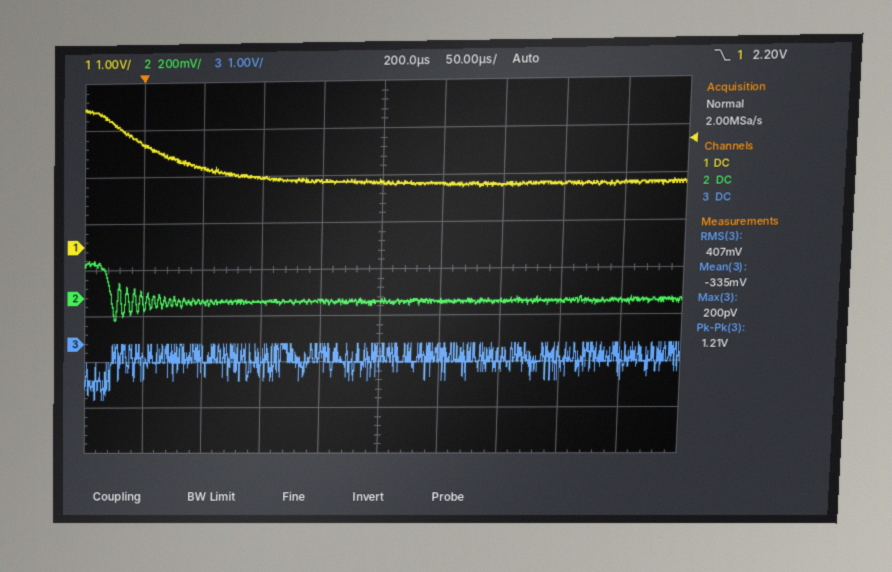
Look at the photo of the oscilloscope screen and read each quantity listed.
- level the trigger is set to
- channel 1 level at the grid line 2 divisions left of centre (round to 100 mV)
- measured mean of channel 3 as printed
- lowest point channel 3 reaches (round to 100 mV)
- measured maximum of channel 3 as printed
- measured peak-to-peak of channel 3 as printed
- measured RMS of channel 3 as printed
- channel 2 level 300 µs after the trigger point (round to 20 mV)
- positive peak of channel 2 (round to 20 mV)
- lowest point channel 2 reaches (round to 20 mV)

2.20 V
1.5 V
-335 mV
-1.2 V
200 pV
1.21 V
407 mV
-20 mV
160 mV
-100 mV
